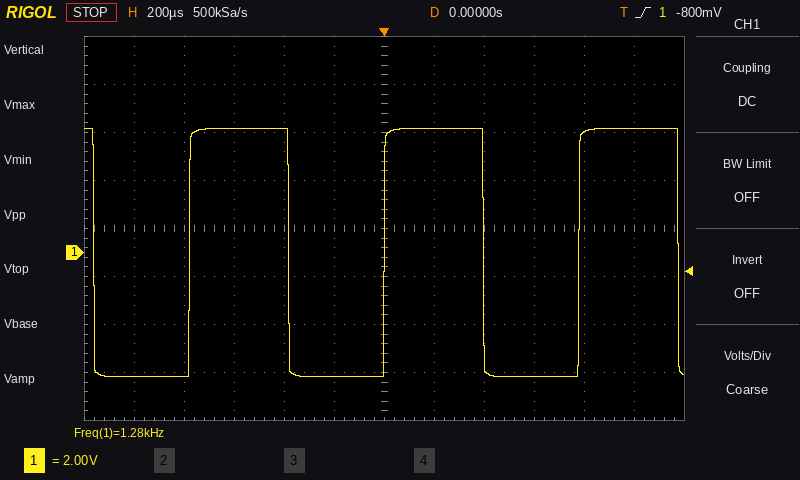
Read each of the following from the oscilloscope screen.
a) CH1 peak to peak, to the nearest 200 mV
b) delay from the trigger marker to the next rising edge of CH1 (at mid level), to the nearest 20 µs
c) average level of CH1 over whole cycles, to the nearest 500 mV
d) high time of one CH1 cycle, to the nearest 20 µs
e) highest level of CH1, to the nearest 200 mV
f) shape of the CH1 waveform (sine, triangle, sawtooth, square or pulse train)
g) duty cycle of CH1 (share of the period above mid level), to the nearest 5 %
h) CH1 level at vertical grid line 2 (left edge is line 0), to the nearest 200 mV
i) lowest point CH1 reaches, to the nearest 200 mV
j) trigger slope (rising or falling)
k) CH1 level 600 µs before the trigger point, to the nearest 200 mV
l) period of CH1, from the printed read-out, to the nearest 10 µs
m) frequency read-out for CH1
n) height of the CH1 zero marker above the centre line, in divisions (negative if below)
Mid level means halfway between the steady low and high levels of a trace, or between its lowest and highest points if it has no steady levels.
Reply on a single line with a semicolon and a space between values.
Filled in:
10.4 V; 780 µs; 0.0 V; 400 µs; 5.2 V; square; 50 %; -5.2 V; -5.2 V; rising; 5.2 V; 780 µs; 1.28 kHz; -0.5 div
